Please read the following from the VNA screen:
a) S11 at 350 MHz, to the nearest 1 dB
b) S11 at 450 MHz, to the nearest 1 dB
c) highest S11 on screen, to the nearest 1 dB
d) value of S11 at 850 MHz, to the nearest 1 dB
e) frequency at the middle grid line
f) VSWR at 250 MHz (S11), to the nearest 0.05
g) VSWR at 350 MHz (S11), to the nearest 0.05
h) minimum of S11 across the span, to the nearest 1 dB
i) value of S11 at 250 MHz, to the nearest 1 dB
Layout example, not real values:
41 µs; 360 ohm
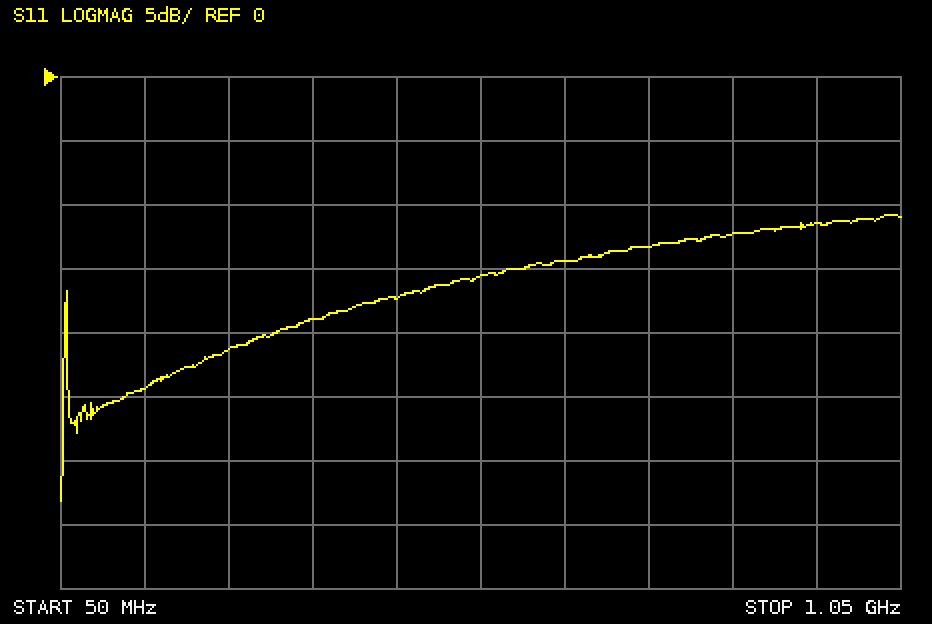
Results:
-19 dB; -17 dB; -11 dB; -12 dB; 550 MHz; 1.20; 1.25; -33 dB; -21 dB
